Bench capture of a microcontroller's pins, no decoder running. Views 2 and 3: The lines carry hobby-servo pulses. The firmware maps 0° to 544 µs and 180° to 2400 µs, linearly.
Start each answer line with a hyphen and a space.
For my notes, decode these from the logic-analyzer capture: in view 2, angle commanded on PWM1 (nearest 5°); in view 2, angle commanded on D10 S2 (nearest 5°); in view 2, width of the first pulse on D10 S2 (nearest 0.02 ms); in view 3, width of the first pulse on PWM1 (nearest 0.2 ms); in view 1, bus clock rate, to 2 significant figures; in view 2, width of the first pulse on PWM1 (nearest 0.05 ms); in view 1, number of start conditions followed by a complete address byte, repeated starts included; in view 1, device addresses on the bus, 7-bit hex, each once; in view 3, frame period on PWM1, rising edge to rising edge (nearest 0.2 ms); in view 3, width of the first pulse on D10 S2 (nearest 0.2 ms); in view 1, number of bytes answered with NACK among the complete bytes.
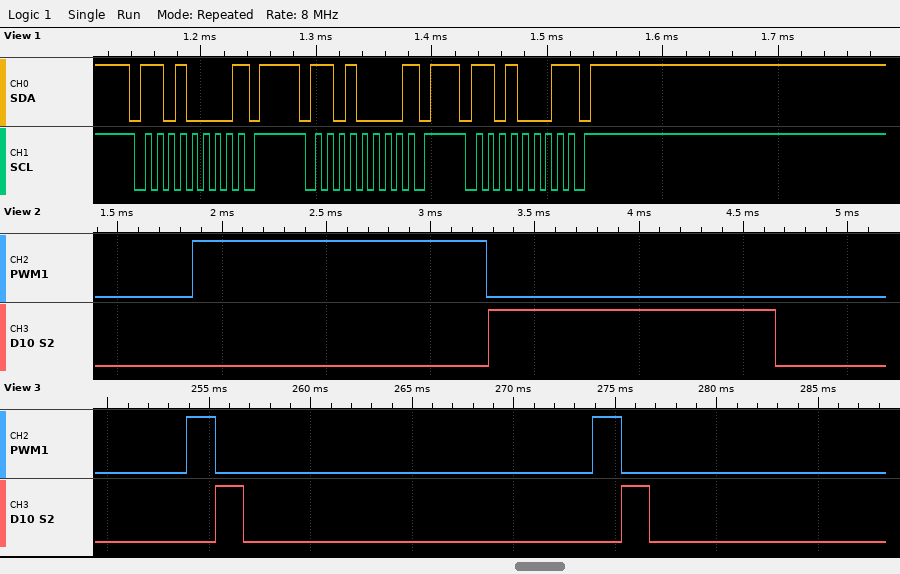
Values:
- 85°
- 80°
- 1.38 ms
- 1.4 ms
- 100 kHz
- 1.40 ms
- 3
- 0x68
- 20.0 ms
- 1.4 ms
- 3
